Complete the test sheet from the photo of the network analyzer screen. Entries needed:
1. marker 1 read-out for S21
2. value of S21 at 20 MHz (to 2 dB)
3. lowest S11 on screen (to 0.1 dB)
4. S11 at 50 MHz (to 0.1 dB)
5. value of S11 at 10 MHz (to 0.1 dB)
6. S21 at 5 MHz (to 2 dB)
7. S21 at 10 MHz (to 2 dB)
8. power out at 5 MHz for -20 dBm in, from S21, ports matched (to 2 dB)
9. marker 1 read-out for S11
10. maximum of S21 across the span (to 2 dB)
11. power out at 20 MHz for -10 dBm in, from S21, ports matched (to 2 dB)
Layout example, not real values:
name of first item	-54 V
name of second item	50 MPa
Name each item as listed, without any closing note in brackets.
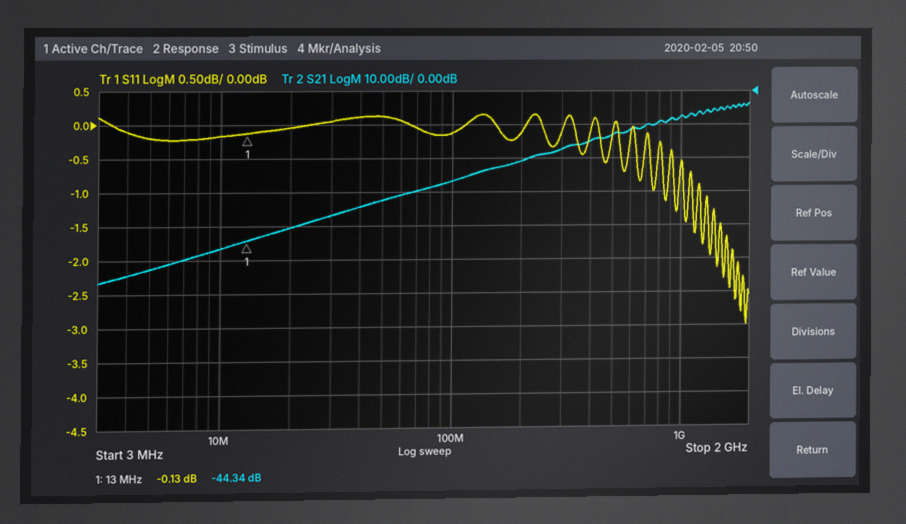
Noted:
marker 1 read-out for S21	-44.34 dB
value of S21 at 20 MHz	-40 dB
lowest S11 on screen	-3.0 dB
S11 at 50 MHz	0.1 dB
value of S11 at 10 MHz	-0.2 dB
S21 at 5 MHz	-52 dB
S21 at 10 MHz	-46 dB
power out at 5 MHz for -20 dBm in, from S21, ports matched	-72 dBm
marker 1 read-out for S11	-0.13 dB
maximum of S21 across the span	-4 dB
power out at 20 MHz for -10 dBm in, from S21, ports matched	-50 dBm
